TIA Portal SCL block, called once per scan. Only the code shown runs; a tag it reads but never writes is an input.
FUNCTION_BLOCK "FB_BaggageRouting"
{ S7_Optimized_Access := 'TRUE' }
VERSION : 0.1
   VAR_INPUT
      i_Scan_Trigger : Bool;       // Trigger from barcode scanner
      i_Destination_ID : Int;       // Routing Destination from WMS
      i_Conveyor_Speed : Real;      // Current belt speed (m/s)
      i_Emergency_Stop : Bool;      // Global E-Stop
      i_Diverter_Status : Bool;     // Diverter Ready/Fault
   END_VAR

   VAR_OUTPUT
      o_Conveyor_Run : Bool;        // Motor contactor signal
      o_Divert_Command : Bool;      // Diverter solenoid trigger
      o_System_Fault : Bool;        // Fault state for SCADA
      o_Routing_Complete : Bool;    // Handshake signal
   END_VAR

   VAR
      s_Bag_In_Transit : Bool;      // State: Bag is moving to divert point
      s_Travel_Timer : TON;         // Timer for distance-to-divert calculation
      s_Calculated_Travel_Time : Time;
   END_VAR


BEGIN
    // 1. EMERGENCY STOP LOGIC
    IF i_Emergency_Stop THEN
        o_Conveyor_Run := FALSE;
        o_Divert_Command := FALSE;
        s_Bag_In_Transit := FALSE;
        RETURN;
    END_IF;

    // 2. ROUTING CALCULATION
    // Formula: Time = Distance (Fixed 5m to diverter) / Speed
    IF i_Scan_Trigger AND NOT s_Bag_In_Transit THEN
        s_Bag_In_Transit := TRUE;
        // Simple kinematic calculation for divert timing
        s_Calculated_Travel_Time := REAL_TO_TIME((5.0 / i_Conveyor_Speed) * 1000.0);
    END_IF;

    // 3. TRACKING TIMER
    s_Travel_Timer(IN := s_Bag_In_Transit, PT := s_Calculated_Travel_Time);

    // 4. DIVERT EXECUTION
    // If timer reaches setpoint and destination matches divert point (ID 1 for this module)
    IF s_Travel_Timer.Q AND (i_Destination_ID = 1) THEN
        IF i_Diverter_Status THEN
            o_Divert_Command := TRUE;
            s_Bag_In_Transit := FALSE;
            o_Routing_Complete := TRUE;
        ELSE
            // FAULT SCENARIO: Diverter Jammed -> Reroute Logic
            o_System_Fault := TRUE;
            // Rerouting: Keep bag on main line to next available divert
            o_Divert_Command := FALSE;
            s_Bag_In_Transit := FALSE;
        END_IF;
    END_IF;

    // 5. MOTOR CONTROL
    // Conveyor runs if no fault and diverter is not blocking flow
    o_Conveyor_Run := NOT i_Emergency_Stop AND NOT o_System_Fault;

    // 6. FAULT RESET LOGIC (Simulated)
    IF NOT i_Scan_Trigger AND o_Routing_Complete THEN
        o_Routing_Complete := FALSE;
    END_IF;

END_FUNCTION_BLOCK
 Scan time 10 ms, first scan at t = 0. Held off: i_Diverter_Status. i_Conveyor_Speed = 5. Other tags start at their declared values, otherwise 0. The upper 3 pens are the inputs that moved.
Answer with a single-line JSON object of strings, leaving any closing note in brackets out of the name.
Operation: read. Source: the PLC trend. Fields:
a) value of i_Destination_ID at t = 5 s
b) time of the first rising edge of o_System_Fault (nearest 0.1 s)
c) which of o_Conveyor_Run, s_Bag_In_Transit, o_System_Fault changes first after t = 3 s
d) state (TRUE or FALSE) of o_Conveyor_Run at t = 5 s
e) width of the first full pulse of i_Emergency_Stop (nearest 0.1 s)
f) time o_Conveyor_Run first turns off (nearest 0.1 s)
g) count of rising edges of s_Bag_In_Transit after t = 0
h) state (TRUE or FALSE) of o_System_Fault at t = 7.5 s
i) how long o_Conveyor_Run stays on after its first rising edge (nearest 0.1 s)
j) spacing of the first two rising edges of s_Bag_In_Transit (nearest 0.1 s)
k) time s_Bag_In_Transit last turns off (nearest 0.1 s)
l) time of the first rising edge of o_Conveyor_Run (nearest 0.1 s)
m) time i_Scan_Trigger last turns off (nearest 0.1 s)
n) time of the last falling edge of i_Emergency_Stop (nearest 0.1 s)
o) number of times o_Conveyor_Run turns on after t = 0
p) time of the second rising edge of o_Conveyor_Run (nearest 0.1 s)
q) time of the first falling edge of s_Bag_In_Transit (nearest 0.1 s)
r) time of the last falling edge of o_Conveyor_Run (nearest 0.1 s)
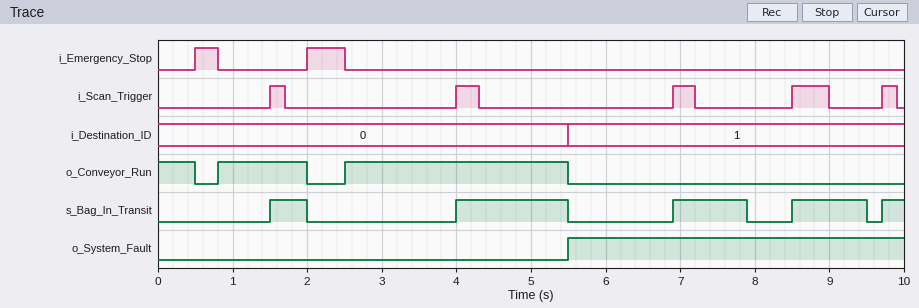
{"value of i_Destination_ID at t = 5 s": "0", "time of the first rising edge of o_System_Fault": "5.5 s", "which of o_Conveyor_Run, s_Bag_In_Transit, o_System_Fault changes first after t = 3 s": "s_Bag_In_Transit", "state (TRUE or FALSE) of o_Conveyor_Run at t = 5 s": "TRUE", "width of the first full pulse of i_Emergency_Stop": "0.3 s", "time o_Conveyor_Run first turns off": "0.5 s", "count of rising edges of s_Bag_In_Transit after t = 0": "5", "state (TRUE or FALSE) of o_System_Fault at t = 7.5 s": "TRUE", "how long o_Conveyor_Run stays on after its first rising edge": "1.2 s", "spacing of the first two rising edges of s_Bag_In_Transit": "2.5 s", "time s_Bag_In_Transit last turns off": "9.5 s", "time of the first rising edge of o_Conveyor_Run": "0.8 s", "time i_Scan_Trigger last turns off": "9.9 s", "time of the last falling edge of i_Emergency_Stop": "2.5 s", "number of times o_Conveyor_Run turns on after t = 0": "2", "time of the second rising edge of o_Conveyor_Run": "2.5 s", "time of the first falling edge of s_Bag_In_Transit": "2.0 s", "time of the last falling edge of o_Conveyor_Run": "5.5 s"}
